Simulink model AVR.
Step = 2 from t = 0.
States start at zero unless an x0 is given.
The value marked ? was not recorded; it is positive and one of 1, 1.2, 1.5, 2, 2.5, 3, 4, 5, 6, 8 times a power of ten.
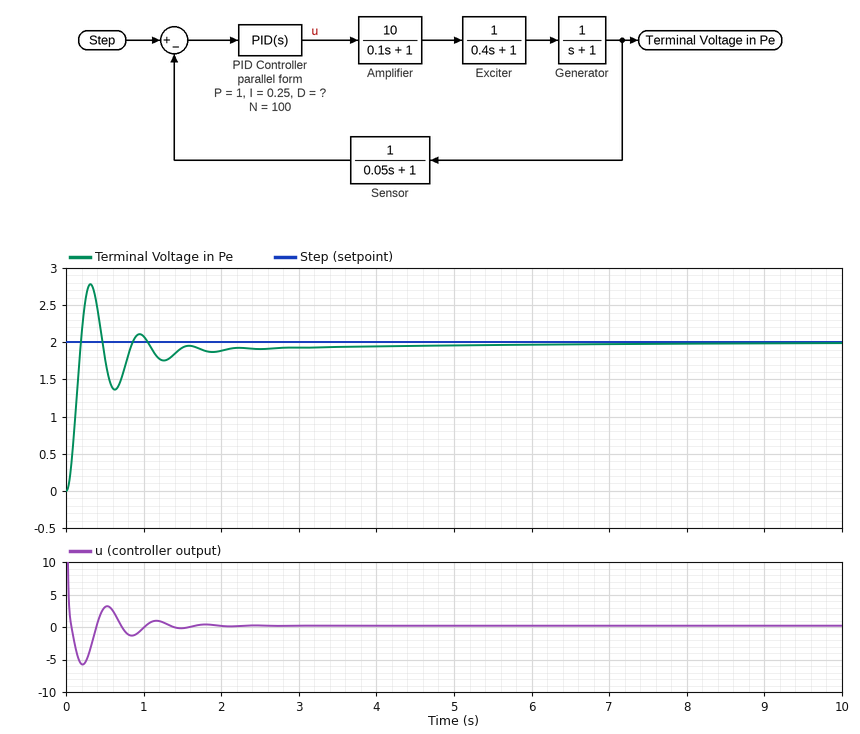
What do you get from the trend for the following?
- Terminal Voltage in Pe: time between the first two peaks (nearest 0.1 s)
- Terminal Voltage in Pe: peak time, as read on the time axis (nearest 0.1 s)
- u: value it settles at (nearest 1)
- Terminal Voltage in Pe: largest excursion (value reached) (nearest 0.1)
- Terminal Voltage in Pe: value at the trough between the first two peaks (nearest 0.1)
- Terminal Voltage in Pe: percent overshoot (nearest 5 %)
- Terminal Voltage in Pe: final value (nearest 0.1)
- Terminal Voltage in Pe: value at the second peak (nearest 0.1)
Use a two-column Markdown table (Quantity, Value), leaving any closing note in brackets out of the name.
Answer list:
| Quantity | Value |
|---|---|
| Terminal Voltage in Pe: time between the first two peaks | 0.6 s |
| Terminal Voltage in Pe: peak time, as read on the time axis | 0.3 s |
| u: value it settles at | 0 |
| Terminal Voltage in Pe: largest excursion (value reached) | 2.8 |
| Terminal Voltage in Pe: value at the trough between the first two peaks | 1.4 |
| Terminal Voltage in Pe: percent overshoot | 40 % |
| Terminal Voltage in Pe: final value | 2.0 |
| Terminal Voltage in Pe: value at the second peak | 2.1 |
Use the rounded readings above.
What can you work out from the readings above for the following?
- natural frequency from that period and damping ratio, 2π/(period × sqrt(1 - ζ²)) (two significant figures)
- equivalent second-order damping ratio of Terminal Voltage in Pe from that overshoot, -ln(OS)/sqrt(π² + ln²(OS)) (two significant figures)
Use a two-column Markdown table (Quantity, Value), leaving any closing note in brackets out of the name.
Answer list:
| Quantity | Value |
|---|---|
| natural frequency from that period and damping ratio, 2π/(period × sqrt(1 - ζ²)) | 11 rad/s |
| equivalent second-order damping ratio of Terminal Voltage in Pe from that overshoot, -ln(OS)/sqrt(π² + ln²(OS)) | 0.28 |
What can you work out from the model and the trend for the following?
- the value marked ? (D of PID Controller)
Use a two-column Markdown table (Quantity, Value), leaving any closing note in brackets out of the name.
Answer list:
| Quantity | Value |
|---|---|
| the value marked ? | 0.5 |
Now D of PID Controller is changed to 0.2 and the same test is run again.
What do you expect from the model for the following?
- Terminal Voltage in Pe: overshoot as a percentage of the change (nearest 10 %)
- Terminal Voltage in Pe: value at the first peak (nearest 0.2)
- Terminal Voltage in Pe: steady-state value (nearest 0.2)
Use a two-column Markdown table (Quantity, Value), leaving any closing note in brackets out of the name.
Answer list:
| Quantity | Value |
|---|---|
| Terminal Voltage in Pe: overshoot as a percentage of the change | 30 % |
| Terminal Voltage in Pe: value at the first peak | 2.6 |
| Terminal Voltage in Pe: steady-state value | 2.0 |
